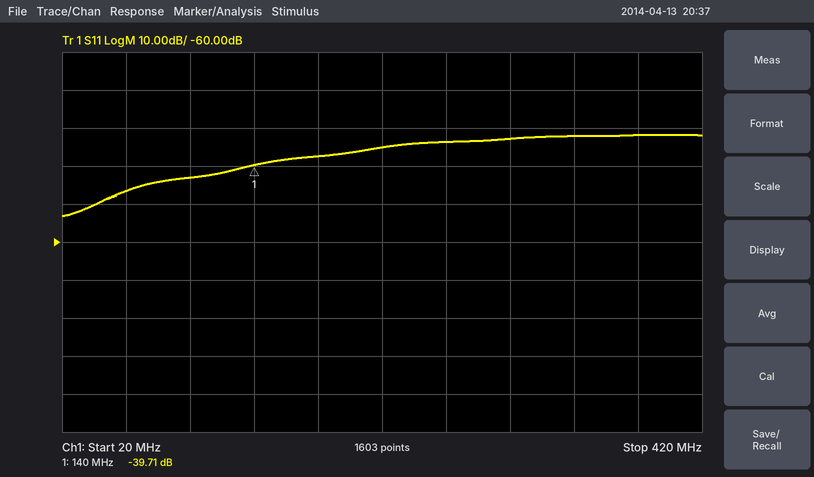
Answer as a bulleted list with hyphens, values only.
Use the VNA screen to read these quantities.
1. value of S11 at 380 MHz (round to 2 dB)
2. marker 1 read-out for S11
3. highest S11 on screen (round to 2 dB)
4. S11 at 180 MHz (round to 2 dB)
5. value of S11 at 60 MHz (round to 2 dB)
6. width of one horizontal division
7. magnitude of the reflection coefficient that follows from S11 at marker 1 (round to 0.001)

- -32 dB
- -39.71 dB
- -32 dB
- -38 dB
- -46 dB
- 40 MHz
- 0.010
